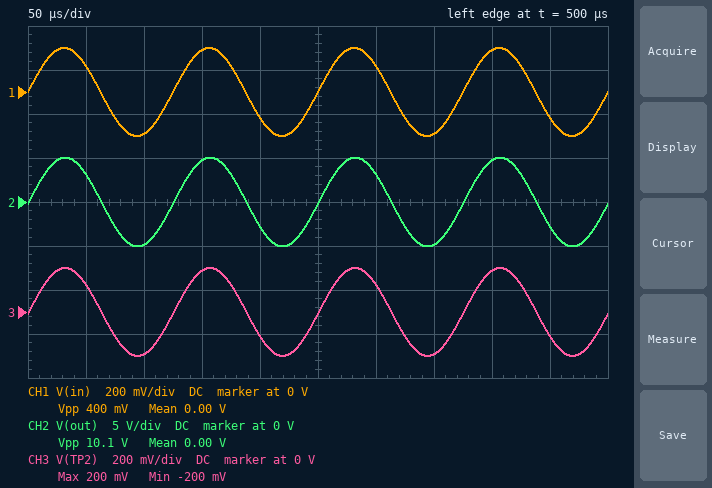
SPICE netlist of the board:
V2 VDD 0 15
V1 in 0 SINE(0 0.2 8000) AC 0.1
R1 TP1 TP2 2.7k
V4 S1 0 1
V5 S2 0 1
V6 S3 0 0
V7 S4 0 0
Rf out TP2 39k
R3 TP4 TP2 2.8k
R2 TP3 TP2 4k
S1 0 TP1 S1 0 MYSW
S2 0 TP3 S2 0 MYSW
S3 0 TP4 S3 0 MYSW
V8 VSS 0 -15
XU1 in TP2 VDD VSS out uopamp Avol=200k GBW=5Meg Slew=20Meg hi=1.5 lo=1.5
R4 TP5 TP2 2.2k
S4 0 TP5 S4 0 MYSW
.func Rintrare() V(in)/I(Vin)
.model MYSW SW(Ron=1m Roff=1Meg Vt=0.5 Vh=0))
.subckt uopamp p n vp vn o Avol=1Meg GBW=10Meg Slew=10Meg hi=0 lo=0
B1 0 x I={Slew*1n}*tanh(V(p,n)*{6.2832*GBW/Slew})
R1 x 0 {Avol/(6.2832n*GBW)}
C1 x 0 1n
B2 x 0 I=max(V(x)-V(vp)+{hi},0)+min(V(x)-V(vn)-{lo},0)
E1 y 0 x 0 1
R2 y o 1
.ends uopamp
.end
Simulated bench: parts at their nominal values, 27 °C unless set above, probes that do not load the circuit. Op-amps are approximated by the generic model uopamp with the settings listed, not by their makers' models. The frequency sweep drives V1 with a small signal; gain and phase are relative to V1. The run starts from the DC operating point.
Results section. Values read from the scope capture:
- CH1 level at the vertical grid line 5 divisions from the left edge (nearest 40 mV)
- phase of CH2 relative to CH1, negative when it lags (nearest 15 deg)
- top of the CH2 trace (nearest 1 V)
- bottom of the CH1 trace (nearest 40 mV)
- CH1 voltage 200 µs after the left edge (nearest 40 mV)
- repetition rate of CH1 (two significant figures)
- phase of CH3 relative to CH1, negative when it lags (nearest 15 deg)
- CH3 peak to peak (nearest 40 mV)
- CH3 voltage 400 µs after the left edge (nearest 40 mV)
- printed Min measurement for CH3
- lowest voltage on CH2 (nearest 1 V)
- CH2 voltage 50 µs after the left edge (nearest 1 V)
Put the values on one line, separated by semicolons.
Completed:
0 V; 0 deg; 5 V; -200 mV; -120 mV; 8.0 kHz; 0 deg; 400 mV; 200 mV; -200 mV; -5 V; 3 V
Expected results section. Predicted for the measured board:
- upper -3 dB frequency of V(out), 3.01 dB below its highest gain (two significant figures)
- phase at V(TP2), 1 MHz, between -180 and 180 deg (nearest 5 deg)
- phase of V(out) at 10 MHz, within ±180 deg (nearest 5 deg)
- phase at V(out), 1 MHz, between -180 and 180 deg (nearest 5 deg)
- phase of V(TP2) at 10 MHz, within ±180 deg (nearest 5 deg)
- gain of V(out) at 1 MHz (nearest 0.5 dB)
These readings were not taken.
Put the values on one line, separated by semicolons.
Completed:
4.3 MHz; -15 deg; -65 deg; -15 deg; -65 deg; 1.0 dB
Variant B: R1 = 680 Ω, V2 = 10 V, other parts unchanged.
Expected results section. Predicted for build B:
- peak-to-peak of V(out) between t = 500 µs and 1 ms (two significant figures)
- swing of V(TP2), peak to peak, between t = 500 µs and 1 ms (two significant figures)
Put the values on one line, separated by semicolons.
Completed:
22 V; 320 mV
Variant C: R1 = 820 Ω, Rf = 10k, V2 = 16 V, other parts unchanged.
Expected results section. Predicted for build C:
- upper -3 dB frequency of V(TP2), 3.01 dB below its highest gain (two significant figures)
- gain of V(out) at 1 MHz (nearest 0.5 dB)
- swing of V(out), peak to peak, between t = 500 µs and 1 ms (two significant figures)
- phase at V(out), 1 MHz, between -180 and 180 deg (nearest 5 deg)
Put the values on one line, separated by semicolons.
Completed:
4.8 MHz; 0 dB; 6.3 V; -10 deg
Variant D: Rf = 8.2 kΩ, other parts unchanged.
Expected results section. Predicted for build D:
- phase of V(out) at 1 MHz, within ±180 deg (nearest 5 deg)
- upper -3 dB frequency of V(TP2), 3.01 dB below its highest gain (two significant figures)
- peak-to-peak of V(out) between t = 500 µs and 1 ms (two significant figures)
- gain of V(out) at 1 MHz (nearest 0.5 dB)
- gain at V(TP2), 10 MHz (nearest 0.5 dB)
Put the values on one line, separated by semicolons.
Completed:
-10 deg; 4.8 MHz; 2.4 V; 0 dB; -7.0 dB
